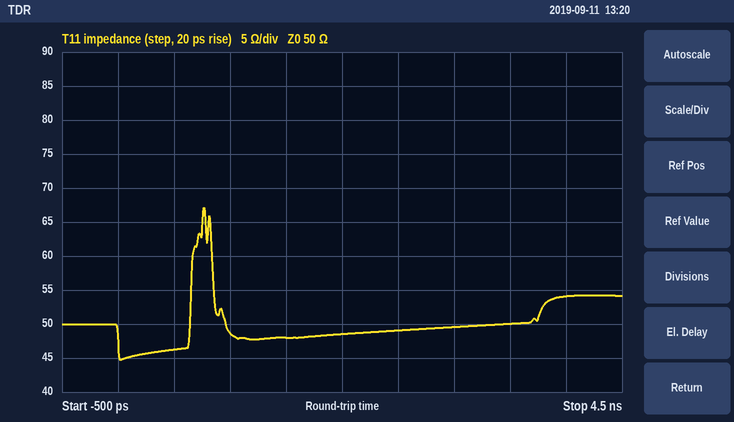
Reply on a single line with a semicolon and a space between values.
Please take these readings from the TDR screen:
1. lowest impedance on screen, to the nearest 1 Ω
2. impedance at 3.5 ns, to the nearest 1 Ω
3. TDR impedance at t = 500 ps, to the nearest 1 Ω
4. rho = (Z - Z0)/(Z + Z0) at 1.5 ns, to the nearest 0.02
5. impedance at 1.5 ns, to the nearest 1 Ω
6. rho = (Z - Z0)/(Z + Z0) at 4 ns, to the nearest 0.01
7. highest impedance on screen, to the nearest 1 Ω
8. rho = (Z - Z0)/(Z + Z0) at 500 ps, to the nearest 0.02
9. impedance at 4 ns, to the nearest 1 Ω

45 Ω; 50 Ω; 46 Ω; -0.02; 48 Ω; +0.04; 67 Ω; -0.04; 54 Ω
